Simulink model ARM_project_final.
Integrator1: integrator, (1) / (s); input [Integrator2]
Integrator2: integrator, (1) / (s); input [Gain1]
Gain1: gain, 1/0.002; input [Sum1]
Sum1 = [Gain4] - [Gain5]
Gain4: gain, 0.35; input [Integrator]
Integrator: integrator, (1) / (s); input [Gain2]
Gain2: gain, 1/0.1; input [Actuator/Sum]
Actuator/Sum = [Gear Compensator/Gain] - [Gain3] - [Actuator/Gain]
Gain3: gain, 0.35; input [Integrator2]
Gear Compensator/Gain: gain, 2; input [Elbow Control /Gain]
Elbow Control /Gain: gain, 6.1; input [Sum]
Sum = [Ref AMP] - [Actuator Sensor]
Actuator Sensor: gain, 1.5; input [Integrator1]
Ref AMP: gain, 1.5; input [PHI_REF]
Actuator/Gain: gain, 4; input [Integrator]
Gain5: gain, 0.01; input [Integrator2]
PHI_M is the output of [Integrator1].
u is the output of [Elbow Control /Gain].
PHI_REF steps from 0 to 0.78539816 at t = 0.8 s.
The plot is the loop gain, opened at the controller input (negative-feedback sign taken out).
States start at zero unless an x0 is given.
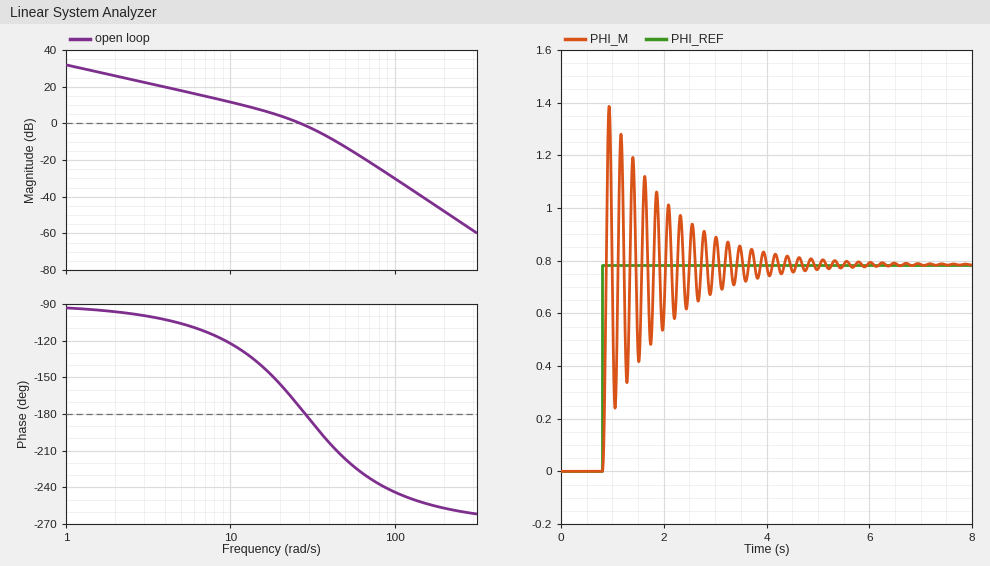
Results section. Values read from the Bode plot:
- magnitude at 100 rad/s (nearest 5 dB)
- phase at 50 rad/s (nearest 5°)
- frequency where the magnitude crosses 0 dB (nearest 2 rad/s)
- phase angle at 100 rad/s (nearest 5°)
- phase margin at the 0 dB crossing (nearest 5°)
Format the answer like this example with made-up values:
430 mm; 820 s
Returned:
-30 dB; -215°; 26 rad/s; -245°; 5°
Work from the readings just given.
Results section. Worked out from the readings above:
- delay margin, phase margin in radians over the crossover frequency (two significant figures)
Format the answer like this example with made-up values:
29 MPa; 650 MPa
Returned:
0.0034 s
